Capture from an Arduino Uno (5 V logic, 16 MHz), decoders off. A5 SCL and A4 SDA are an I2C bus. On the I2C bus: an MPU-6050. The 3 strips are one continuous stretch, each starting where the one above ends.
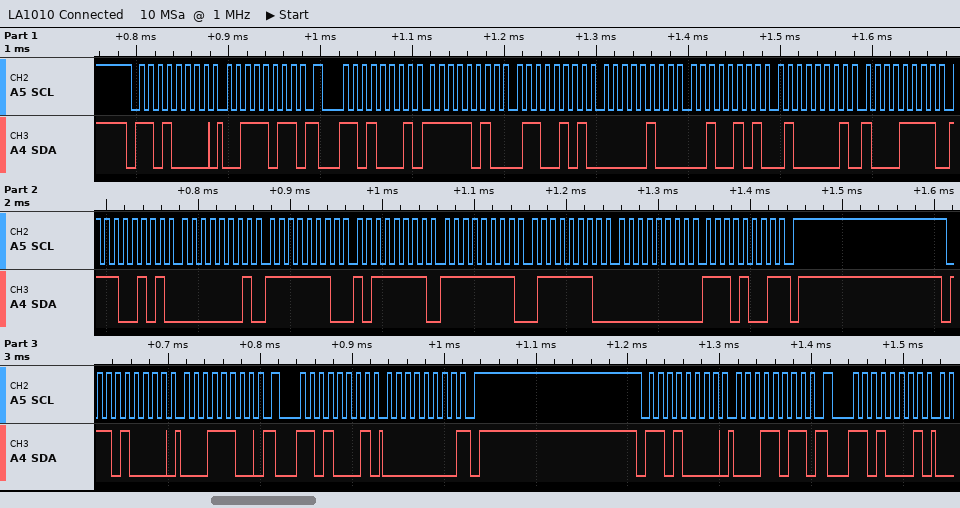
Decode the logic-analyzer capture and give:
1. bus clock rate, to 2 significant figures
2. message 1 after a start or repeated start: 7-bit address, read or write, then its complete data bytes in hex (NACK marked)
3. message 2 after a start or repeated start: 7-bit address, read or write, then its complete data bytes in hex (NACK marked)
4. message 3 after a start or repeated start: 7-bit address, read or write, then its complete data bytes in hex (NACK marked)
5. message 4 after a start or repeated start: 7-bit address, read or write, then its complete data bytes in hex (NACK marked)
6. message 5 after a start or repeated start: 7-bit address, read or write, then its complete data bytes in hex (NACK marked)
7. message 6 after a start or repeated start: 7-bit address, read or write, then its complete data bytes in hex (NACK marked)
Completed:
100 kHz
0x68 write: 3B
0x68 read: FA 65 04 25 41 8F E5 01 FE BF FF 7E 00 E9 NACK
0x68 write: 1C
0x68 read: 00 NACK
0x68 write: 1B
0x68 read
